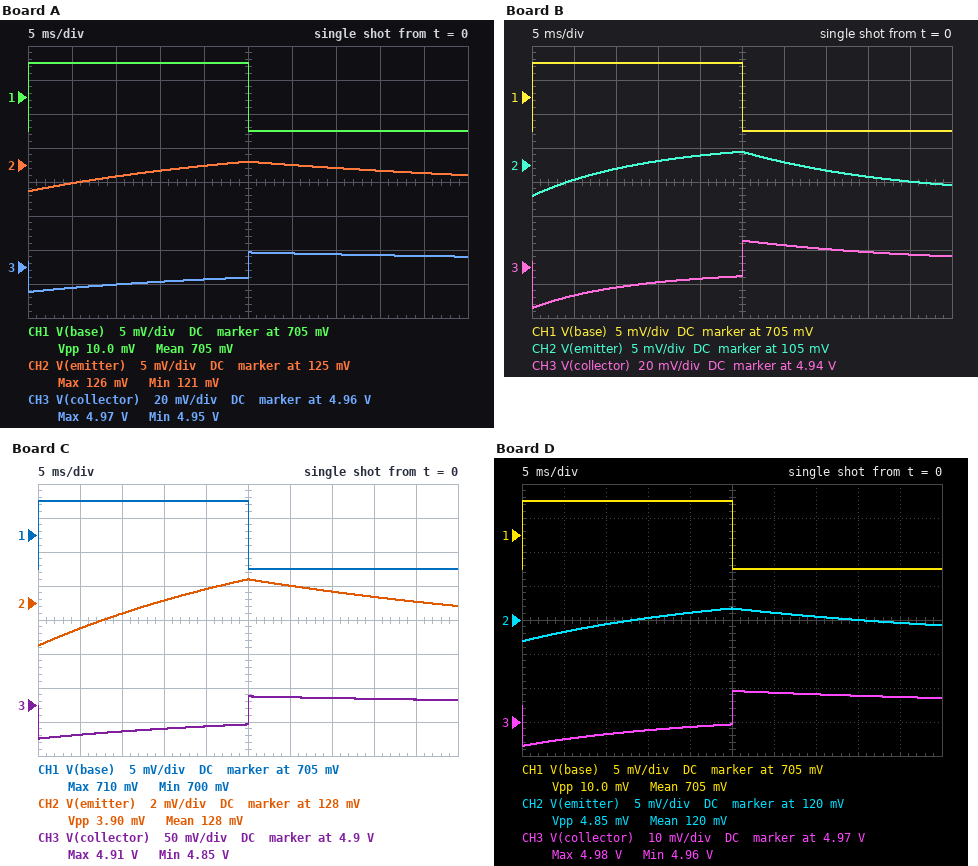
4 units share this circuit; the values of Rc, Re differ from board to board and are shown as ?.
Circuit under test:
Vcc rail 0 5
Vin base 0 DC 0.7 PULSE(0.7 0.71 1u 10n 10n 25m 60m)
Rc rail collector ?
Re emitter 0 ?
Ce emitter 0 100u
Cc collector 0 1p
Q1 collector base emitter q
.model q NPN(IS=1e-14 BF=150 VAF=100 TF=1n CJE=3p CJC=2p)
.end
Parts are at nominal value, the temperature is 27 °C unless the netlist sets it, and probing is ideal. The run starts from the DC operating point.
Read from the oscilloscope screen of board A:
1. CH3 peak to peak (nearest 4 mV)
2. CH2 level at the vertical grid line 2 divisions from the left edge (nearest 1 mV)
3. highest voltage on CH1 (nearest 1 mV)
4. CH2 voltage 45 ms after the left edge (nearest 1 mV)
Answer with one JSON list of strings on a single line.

["24 mV", "123 mV", "710 mV", "124 mV"]
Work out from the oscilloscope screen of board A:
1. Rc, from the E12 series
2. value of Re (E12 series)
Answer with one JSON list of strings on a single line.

["680 Ω", "2.2 kΩ"]
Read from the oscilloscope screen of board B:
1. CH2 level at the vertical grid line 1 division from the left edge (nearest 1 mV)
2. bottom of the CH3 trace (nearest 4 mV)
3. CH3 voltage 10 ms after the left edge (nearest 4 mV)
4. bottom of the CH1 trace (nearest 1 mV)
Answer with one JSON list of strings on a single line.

["103 mV", "4.916 V", "4.928 V", "700 mV"]
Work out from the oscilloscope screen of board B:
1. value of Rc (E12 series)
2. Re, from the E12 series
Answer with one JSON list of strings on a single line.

["470 Ω", "820 Ω"]
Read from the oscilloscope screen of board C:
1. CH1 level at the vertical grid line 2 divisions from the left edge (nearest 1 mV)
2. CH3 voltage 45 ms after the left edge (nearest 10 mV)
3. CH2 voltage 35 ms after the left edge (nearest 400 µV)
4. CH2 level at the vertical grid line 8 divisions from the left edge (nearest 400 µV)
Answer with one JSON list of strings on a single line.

["710 mV", "4.91 V", "128.8 mV", "128.4 mV"]
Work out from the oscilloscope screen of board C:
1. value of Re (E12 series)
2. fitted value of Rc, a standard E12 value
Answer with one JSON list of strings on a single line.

["2.7 kΩ", "2.2 kΩ"]
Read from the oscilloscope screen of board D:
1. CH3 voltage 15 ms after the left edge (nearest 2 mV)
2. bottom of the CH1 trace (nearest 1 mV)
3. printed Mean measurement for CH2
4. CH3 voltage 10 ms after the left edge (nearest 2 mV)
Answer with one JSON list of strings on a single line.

["4.968 V", "700 mV", "120 mV", "4.966 V"]
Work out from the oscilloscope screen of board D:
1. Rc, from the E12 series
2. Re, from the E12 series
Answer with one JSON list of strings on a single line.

["390 Ω", "1.8 kΩ"]
